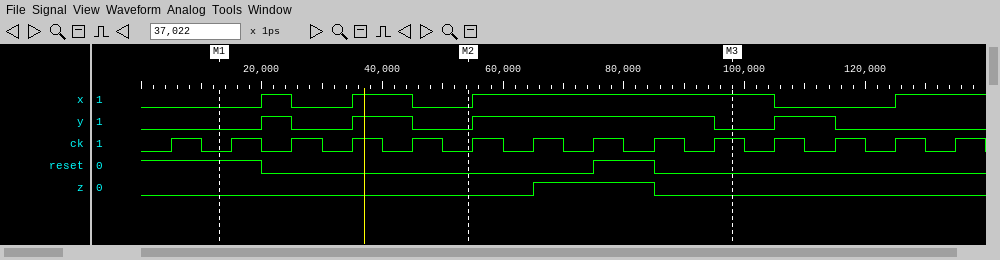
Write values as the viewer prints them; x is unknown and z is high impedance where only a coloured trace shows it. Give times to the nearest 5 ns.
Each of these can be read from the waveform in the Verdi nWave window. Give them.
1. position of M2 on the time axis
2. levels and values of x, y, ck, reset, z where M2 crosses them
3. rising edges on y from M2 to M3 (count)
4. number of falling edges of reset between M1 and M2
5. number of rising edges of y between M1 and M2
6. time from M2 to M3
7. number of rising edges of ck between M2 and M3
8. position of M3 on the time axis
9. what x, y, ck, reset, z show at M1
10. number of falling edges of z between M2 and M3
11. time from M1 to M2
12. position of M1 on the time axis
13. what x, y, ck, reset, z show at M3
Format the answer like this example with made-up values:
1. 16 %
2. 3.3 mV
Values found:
1. 55 ns
2. x=0, y=0, ck=0, reset=0, z=0
3. 1
4. 1
5. 2
6. 45 ns
7. 5
8. 100 ns
9. x=0, y=0, ck=0, reset=1, z=0
10. 1
11. 40 ns
12. 15 ns
13. x=1, y=0, ck=1, reset=0, z=0
